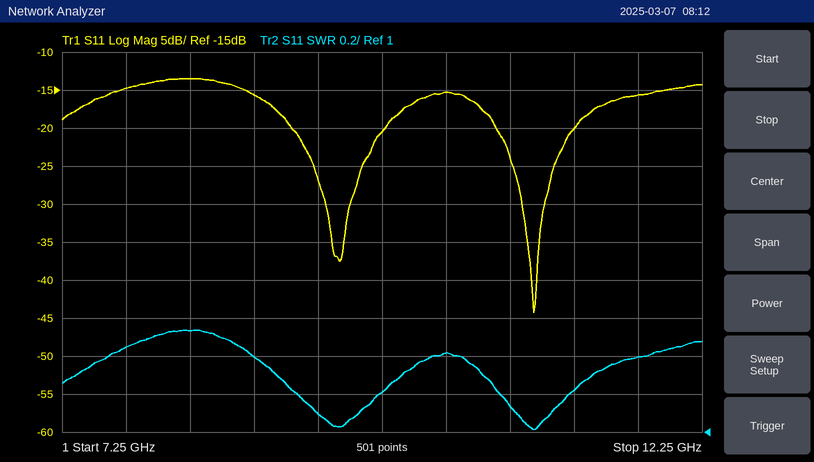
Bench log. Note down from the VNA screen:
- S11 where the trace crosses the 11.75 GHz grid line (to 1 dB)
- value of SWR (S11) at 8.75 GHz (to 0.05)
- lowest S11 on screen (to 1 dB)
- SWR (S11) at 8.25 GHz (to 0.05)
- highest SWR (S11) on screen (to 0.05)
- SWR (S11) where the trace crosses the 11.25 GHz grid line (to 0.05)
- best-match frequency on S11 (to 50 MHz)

-16 dB
1.40
-44 dB
1.55
1.55
1.20
10.95 GHz
